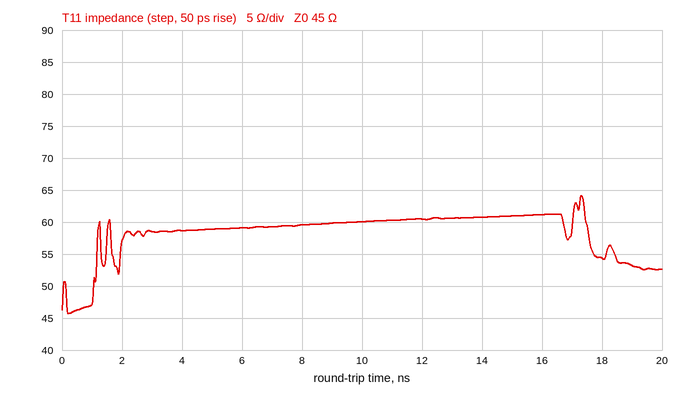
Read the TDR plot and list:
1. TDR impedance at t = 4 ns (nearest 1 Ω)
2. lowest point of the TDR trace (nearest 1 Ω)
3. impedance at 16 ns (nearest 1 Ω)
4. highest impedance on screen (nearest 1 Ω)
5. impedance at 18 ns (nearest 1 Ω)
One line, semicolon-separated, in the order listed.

59 Ω; 46 Ω; 61 Ω; 64 Ω; 54 Ω
